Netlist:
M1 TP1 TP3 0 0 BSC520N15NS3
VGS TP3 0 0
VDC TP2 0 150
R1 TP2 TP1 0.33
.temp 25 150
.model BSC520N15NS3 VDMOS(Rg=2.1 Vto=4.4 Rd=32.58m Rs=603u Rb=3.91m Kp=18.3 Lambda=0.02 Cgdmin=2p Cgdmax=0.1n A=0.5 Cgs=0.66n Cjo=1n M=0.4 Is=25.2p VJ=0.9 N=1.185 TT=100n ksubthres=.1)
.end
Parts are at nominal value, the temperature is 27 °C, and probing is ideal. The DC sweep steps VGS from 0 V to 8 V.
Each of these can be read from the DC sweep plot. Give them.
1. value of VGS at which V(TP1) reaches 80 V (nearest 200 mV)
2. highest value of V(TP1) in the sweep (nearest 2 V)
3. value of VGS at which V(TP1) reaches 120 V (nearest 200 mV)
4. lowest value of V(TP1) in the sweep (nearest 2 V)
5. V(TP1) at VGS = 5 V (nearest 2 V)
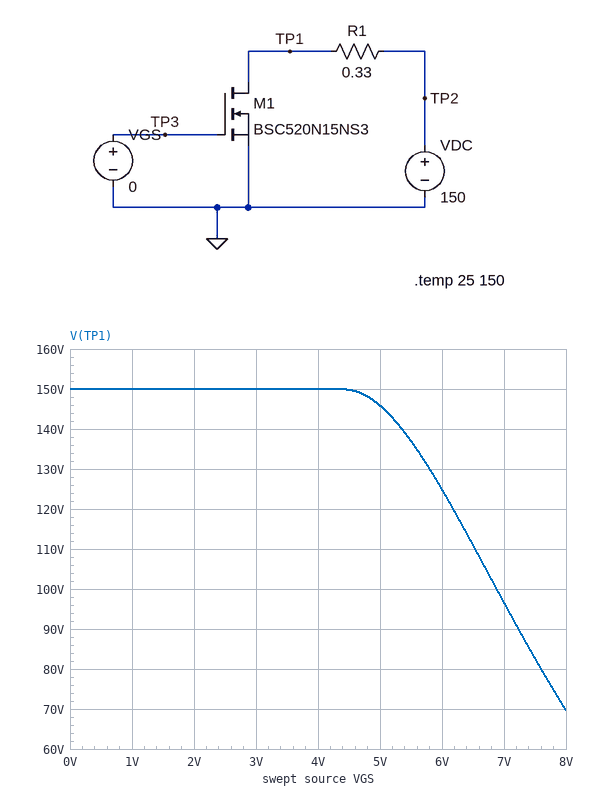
7.6 V
150 V
6.2 V
70 V
146 V
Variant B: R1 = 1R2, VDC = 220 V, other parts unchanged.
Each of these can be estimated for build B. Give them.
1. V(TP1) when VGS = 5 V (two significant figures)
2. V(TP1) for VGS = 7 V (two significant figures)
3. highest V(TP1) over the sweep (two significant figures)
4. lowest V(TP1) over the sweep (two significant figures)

200 V
65 V
220 V
27 V
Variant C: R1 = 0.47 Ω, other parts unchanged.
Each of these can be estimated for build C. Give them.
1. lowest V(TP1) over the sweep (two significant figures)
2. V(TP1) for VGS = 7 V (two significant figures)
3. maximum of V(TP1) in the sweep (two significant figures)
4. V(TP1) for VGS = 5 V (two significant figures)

52 V
81 V
150 V
140 V
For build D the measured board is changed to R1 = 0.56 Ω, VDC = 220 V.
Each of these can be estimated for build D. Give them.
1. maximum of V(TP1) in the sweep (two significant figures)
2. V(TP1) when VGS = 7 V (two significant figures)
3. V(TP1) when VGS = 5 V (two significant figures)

220 V
120 V
210 V
